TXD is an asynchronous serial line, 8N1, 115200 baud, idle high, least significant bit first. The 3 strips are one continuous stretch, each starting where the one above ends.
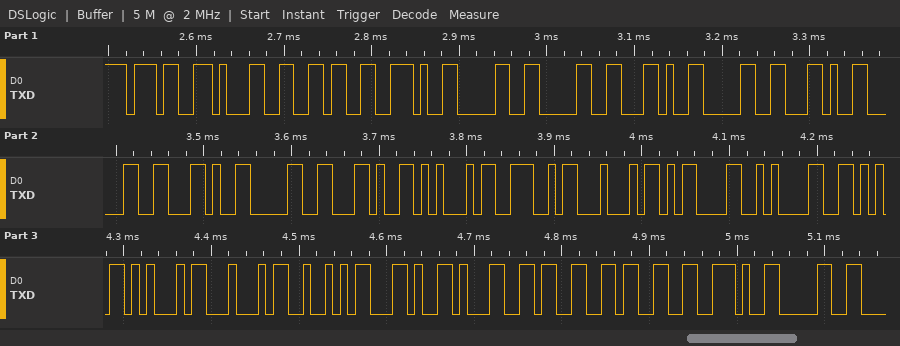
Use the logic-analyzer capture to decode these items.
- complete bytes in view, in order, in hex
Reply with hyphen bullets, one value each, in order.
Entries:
- 0x37 0x31 0x36 0x2E 0x30 0x30 0x2C 0x30 0x2C 0x30 0x2C 0x30 0x2C 0x45 0x4E 0x44 0x0D 0x0A 0x56 0x45 0x44 0x52 0x2C 0x31 0x33 0x33 0x2E 0x30
